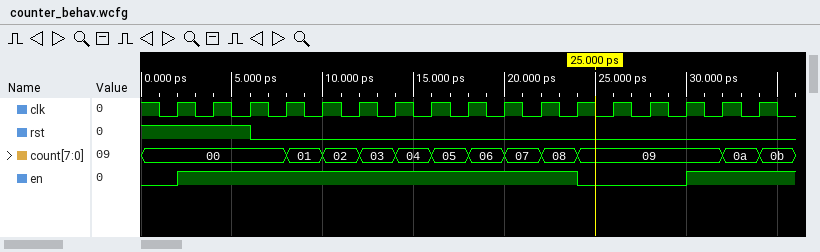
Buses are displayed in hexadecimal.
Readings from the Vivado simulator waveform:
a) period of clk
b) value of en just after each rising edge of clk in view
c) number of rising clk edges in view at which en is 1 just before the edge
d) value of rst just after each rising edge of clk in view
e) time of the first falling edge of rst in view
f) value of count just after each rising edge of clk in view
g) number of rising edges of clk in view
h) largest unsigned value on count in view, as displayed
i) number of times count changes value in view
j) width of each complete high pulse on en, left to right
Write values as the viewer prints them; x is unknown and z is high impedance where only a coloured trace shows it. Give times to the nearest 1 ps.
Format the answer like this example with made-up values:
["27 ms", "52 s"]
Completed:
["2 ps", "1 1 1 1 1 1 1 1 1 1 1 0 0 0 1 1 1", "13", "1 1 0 0 0 0 0 0 0 0 0 0 0 0 0 0 0", "6 ps", "00, 00, 00, 01, 02, 03, 04, 05, 06, 07, 08, 09, 09, 09, 09, 0a, 0b", "17", "0b", "11", "22 ps"]
